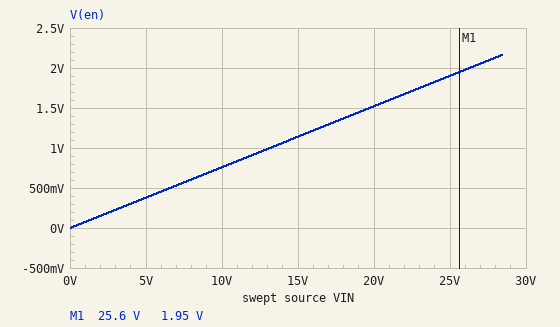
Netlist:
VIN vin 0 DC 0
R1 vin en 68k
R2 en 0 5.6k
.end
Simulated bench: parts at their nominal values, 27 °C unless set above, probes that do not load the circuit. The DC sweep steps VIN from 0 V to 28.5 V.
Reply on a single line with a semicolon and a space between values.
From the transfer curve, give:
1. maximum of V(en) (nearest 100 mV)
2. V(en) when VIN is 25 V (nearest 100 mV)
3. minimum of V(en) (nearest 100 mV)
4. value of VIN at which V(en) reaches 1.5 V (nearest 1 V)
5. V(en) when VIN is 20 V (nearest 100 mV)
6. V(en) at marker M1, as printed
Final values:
2.2 V; 1.9 V; 0 V; 20 V; 1.5 V; 1.95 V
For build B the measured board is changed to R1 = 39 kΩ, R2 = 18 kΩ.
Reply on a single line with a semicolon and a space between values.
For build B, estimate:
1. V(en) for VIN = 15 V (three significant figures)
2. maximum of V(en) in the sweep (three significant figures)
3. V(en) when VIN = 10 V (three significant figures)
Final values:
4.74 V; 9.00 V; 3.16 V
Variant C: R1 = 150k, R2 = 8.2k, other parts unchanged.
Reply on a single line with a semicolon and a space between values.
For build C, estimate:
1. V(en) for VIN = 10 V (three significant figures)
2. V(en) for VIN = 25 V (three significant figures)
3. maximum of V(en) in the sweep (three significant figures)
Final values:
518 mV; 1.30 V; 1.48 V
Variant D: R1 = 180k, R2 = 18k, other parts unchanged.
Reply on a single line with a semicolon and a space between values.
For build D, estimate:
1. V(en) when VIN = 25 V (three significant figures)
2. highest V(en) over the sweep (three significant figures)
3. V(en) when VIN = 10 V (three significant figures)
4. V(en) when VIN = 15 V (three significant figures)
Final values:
2.27 V; 2.59 V; 909 mV; 1.36 V
